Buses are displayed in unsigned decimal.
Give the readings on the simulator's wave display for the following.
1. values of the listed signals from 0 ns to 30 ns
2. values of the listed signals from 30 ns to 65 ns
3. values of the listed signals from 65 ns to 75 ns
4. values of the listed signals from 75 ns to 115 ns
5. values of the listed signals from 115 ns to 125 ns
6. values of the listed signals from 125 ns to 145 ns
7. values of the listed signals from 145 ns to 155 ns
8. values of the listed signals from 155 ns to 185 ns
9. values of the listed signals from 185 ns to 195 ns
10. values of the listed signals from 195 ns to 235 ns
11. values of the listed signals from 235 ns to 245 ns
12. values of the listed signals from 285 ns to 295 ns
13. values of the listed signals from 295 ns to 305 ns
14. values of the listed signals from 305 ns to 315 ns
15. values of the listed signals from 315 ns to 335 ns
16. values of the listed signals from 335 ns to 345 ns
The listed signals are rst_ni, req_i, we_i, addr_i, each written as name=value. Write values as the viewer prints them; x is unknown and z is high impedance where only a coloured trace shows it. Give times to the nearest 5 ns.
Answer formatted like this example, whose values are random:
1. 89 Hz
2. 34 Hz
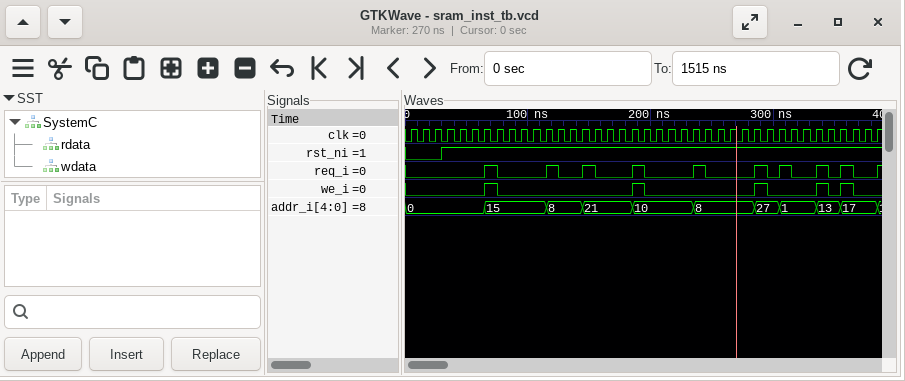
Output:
1. rst_ni=0, req_i=0, we_i=0, addr_i=0
2. rst_ni=1, req_i=0, we_i=0, addr_i=0
3. rst_ni=1, req_i=1, we_i=1, addr_i=15
4. rst_ni=1, req_i=0, we_i=0, addr_i=15
5. rst_ni=1, req_i=1, we_i=0, addr_i=8
6. rst_ni=1, req_i=0, we_i=0, addr_i=8
7. rst_ni=1, req_i=1, we_i=0, addr_i=21
8. rst_ni=1, req_i=0, we_i=0, addr_i=21
9. rst_ni=1, req_i=1, we_i=1, addr_i=10
10. rst_ni=1, req_i=0, we_i=0, addr_i=10
11. rst_ni=1, req_i=1, we_i=0, addr_i=8
12. rst_ni=1, req_i=1, we_i=1, addr_i=27
13. rst_ni=1, req_i=0, we_i=0, addr_i=27
14. rst_ni=1, req_i=1, we_i=0, addr_i=1
15. rst_ni=1, req_i=0, we_i=0, addr_i=1
16. rst_ni=1, req_i=1, we_i=1, addr_i=13
